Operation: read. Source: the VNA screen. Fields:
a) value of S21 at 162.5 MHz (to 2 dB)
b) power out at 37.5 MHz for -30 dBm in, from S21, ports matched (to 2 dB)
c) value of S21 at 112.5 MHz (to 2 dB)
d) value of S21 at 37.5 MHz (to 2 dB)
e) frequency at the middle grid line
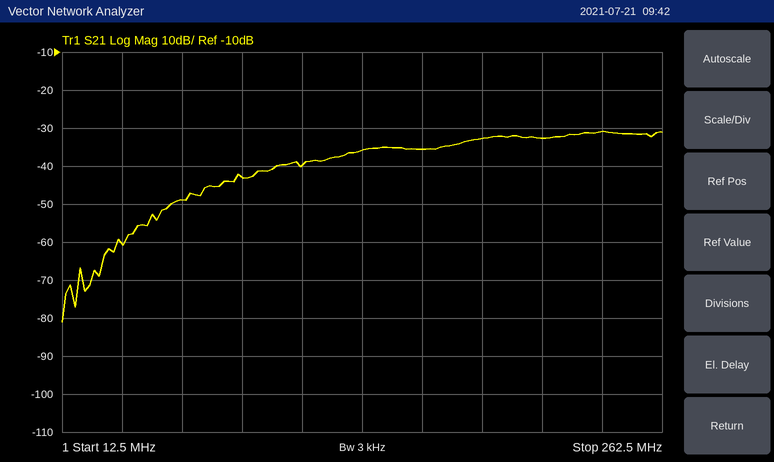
-36 dB
-90 dBm
-40 dB
-60 dB
137.5 MHz
